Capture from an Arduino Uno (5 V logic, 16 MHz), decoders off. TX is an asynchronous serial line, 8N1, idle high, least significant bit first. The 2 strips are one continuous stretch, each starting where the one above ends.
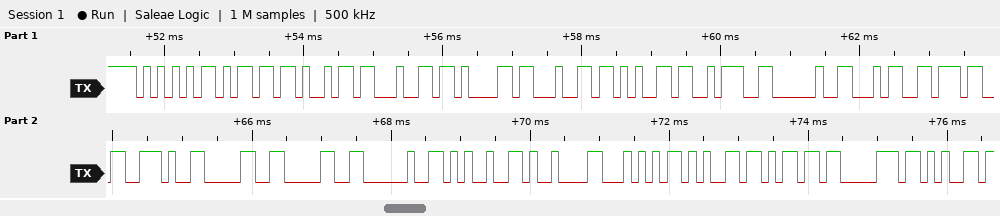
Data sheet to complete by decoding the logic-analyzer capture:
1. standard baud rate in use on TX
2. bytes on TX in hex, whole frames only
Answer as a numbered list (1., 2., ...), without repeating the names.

1. 9600 baud
2. 55 6D 69 64 61 64 65 3A 20 34 37 2E 30 30 20 25 09 54 65 6D 70 65
